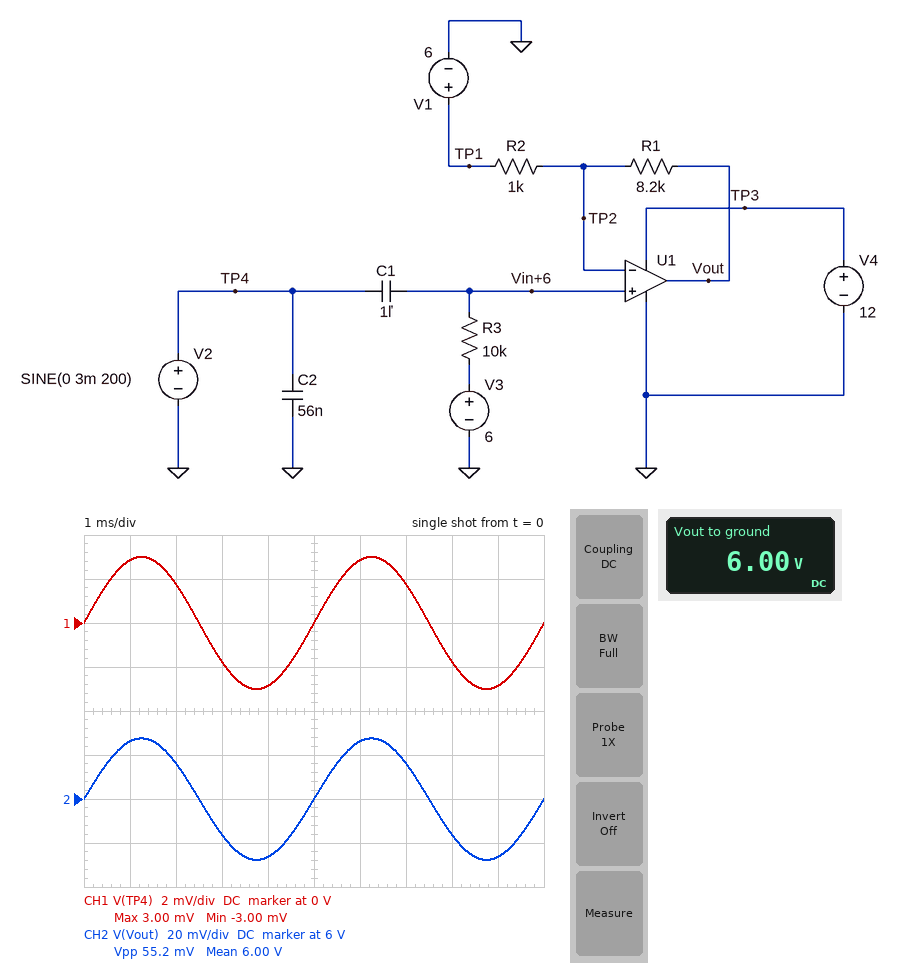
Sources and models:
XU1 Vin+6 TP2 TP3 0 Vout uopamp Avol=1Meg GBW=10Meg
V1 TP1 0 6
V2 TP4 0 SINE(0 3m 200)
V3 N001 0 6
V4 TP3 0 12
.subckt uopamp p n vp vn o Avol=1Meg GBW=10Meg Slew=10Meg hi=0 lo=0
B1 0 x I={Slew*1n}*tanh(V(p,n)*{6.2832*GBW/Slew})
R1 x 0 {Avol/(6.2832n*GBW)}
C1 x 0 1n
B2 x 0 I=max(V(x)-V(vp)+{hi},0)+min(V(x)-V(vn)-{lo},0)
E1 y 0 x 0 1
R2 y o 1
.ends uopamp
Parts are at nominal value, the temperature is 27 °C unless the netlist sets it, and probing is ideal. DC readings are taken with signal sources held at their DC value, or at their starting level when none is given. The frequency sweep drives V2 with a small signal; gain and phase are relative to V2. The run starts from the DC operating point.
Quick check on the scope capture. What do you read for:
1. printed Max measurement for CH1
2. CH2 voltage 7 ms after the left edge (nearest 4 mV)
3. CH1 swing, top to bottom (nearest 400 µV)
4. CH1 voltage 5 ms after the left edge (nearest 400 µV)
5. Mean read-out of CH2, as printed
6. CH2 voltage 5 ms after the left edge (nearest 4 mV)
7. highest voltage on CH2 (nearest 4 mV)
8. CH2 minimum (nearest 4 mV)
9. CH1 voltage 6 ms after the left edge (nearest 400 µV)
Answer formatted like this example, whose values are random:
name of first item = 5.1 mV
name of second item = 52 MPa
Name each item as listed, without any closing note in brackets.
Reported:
printed Max measurement for CH1 = 3.00 mV
CH2 voltage 7 ms after the left edge = 6.016 V
CH1 swing, top to bottom = 6.0 mV
CH1 voltage 5 ms after the left edge = 0 V
Mean read-out of CH2, as printed = 6.00 V
CH2 voltage 5 ms after the left edge = 6.000 V
highest voltage on CH2 = 6.028 V
CH2 minimum = 5.972 V
CH1 voltage 6 ms after the left edge = 2.8 mV
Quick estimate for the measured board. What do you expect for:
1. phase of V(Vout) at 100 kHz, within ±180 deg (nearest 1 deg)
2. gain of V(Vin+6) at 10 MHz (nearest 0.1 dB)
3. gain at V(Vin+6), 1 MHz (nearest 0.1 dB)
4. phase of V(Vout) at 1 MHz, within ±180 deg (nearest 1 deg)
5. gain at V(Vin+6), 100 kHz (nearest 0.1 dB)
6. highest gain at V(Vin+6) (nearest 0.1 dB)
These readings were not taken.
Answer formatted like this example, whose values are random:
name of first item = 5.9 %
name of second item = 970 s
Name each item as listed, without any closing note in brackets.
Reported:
phase of V(Vout) at 100 kHz, within ±180 deg = -5 deg
gain of V(Vin+6) at 10 MHz = 0 dB
gain at V(Vin+6), 1 MHz = 0 dB
phase of V(Vout) at 1 MHz, within ±180 deg = -43 deg
gain at V(Vin+6), 100 kHz = 0 dB
highest gain at V(Vin+6) = 0 dB
